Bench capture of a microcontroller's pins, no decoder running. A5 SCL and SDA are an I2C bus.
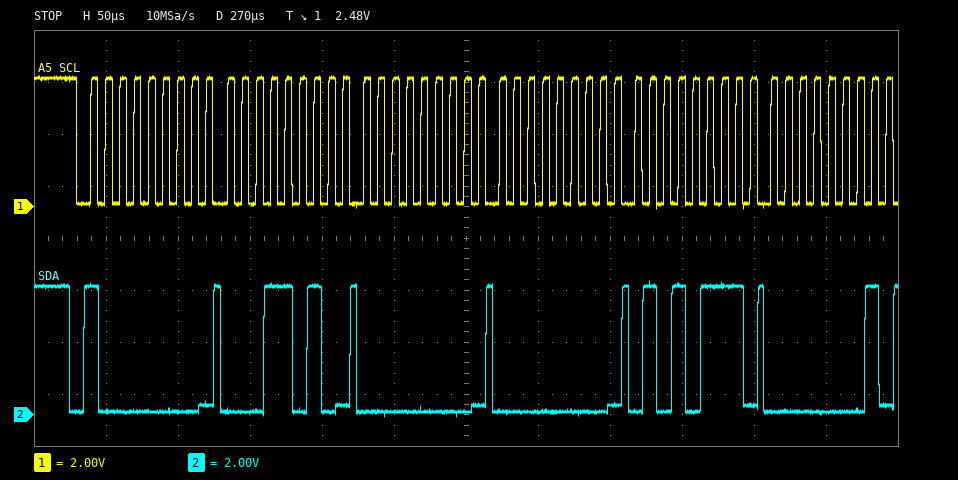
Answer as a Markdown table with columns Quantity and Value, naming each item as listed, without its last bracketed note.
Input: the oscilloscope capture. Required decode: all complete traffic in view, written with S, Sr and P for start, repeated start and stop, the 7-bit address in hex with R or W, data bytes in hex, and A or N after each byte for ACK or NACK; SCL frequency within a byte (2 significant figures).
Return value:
| Quantity | Value |
|---|---|
| all complete traffic in view, written with S, Sr and P for start, repeated start and stop, the 7-bit address in hex with R or W, data bytes in hex, and A or N after each byte for ACK or NACK | S 40W A 1A A 00 A 00 A 57 A 01 A |
| SCL frequency within a byte | 100 kHz |
